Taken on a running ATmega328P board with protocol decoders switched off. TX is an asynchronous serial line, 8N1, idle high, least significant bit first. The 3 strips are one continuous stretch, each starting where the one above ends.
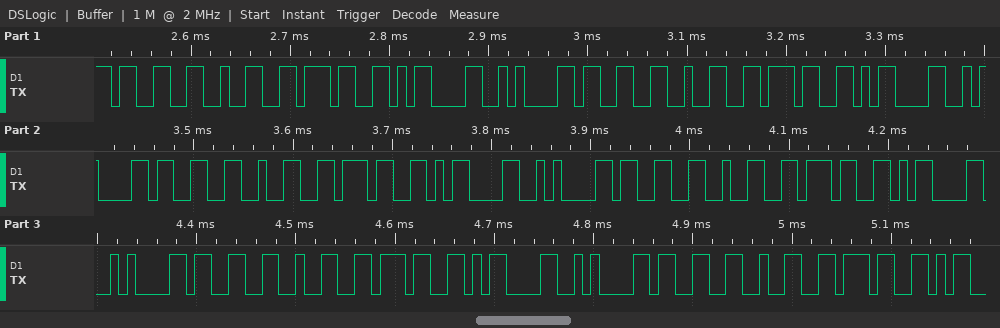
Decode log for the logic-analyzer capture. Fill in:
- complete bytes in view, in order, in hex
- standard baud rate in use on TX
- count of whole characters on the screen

33 32 37 0D 0A 33 32 37 0D 0A 33 32 37 0D 0A 33 32 37 0D 0A 33 32 37 0D 0A 33 32 37
115200 baud
28
